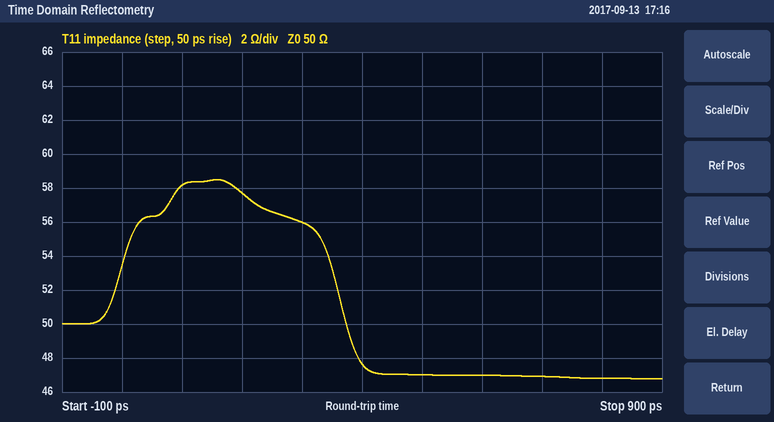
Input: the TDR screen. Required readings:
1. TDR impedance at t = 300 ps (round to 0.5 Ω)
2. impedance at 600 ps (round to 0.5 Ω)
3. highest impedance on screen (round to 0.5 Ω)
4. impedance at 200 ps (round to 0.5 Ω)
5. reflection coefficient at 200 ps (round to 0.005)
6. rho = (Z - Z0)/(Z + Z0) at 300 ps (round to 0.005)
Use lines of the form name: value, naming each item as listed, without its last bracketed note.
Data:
TDR impedance at t = 300 ps: 56.0 Ω
impedance at 600 ps: 47.0 Ω
highest impedance on screen: 58.5 Ω
impedance at 200 ps: 57.5 Ω
reflection coefficient at 200 ps: +0.070
rho = (Z - Z0)/(Z + Z0) at 300 ps: +0.055
